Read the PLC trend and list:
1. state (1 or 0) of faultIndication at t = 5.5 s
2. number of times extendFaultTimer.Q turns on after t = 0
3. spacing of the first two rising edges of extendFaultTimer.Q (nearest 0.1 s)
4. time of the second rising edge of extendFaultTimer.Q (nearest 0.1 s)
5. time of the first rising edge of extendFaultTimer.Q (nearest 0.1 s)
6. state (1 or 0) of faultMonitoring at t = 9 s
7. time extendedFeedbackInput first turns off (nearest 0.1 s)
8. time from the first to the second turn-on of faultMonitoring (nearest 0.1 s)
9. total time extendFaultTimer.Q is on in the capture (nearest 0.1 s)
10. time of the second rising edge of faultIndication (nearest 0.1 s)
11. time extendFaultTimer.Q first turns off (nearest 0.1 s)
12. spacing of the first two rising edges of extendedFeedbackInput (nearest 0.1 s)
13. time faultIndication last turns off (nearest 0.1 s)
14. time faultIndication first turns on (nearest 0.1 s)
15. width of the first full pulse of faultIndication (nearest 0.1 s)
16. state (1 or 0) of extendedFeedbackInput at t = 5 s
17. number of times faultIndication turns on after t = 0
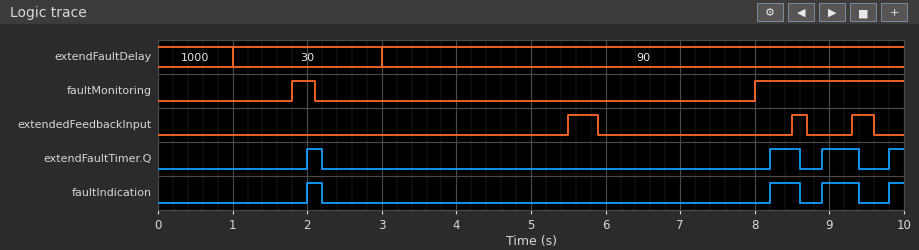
0
4
6.2 s
8.2 s
2.0 s
1
5.9 s
6.2 s
1.3 s
8.2 s
2.2 s
3.0 s
9.4 s
2.0 s
0.2 s
0
4
